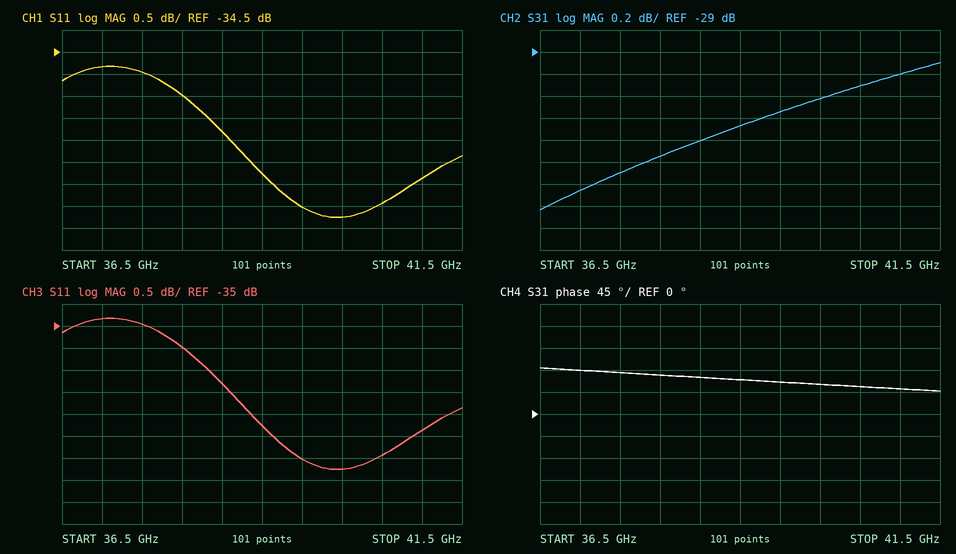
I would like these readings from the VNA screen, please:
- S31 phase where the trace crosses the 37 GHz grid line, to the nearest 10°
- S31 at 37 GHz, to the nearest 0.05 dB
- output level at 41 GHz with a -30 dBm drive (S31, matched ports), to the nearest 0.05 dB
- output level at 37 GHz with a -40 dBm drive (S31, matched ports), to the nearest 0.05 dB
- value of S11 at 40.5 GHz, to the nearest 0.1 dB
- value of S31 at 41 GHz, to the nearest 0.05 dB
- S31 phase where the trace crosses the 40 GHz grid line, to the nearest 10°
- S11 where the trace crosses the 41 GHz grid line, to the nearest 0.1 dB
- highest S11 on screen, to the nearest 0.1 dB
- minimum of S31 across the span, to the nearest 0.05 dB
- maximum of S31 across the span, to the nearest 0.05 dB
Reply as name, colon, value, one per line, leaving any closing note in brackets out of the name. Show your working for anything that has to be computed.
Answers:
S31 phase where the trace crosses the 37 GHz grid line, to the nearest 10°: 90°
S31 at 37 GHz, to the nearest 0.05 dB: -30.25 dB
output level at 41 GHz with a -30 dBm drive (S31, matched ports), to the nearest 0.05 dB: -30 dBm + (-29.20 dB) = -59.20 dBm
output level at 37 GHz with a -40 dBm drive (S31, matched ports), to the nearest 0.05 dB: -40 dBm + (-30.25 dB) = -70.25 dBm
value of S11 at 40.5 GHz, to the nearest 0.1 dB: -37.9 dB
value of S31 at 41 GHz, to the nearest 0.05 dB: -29.20 dB
S31 phase where the trace crosses the 40 GHz grid line, to the nearest 10°: 60°
S11 where the trace crosses the 41 GHz grid line, to the nearest 0.1 dB: -37.4 dB
highest S11 on screen, to the nearest 0.1 dB: -34.8 dB
minimum of S31 across the span, to the nearest 0.05 dB: -30.45 dB
maximum of S31 across the span, to the nearest 0.05 dB: -29.10 dB
